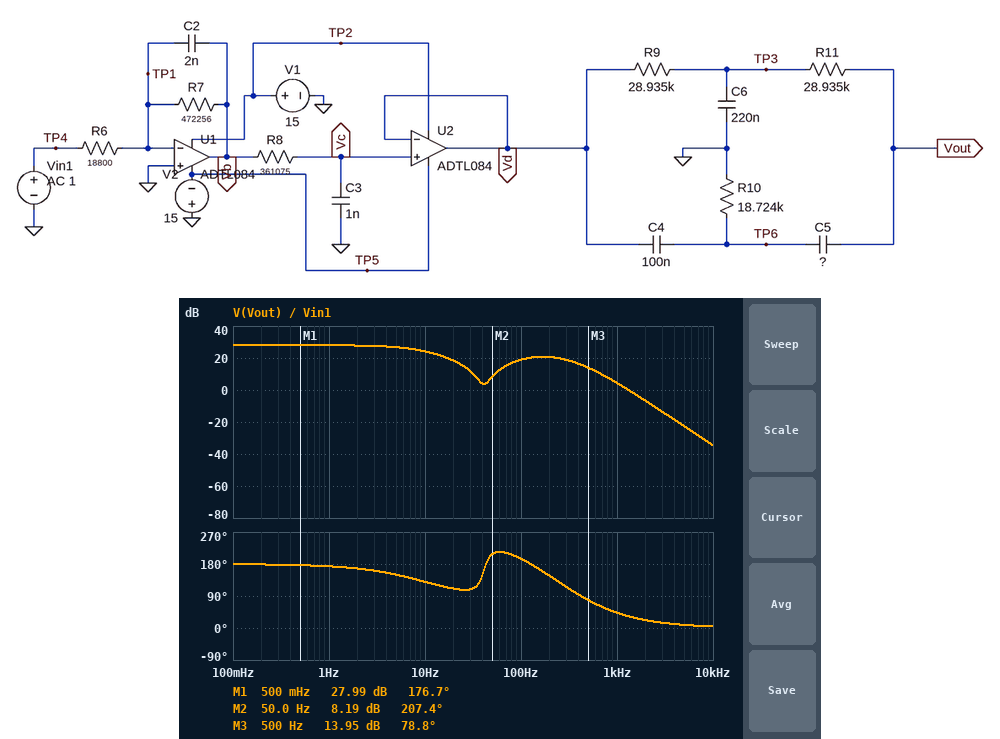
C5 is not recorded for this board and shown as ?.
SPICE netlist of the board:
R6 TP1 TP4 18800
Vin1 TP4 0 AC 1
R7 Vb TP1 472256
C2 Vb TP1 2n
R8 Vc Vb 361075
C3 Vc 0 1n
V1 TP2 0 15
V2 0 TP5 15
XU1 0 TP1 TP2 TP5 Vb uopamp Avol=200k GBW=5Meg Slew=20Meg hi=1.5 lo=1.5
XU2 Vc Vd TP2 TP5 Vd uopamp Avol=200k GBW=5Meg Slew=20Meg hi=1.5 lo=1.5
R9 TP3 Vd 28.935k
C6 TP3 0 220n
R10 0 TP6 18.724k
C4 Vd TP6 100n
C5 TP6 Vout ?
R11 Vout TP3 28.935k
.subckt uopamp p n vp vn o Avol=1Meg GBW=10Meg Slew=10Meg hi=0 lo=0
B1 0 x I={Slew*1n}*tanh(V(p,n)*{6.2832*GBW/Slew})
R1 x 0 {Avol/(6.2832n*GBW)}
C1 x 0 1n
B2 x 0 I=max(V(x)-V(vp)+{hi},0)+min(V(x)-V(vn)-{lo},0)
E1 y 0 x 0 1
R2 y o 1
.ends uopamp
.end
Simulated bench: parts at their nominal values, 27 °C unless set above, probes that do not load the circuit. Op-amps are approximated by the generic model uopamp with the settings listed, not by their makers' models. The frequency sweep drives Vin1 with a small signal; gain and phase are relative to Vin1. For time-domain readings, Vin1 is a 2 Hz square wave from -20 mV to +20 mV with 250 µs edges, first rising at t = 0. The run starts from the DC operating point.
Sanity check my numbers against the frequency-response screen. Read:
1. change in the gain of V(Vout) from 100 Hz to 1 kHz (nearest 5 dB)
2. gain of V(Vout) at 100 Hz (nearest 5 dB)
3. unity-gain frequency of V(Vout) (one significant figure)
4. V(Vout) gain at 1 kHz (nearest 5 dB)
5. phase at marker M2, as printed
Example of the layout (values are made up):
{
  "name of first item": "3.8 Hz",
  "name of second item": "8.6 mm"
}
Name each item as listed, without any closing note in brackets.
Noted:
{
  "change in the gain of V(Vout) from 100 Hz to 1 kHz": "-15 dB",
  "gain of V(Vout) at 100 Hz": "20 dB",
  "unity-gain frequency of V(Vout)": "1 kHz",
  "V(Vout) gain at 1 kHz": "5 dB",
  "phase at marker M2, as printed": "207.4 deg"
}
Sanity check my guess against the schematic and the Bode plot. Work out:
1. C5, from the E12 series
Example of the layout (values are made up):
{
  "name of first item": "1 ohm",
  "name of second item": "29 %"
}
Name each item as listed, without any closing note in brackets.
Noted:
{
  "C5, from the E12 series": "180 nF"
}
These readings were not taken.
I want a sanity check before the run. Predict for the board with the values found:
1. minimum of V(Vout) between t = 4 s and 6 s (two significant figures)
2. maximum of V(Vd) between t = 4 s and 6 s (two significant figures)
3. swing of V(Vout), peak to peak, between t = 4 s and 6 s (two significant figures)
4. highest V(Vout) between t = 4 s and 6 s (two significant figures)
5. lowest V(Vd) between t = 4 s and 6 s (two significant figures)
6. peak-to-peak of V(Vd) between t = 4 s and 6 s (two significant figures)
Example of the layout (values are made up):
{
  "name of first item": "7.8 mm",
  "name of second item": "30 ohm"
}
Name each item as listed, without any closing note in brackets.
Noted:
{
  "minimum of V(Vout) between t = 4 s and 6 s": "-500 mV",
  "maximum of V(Vd) between t = 4 s and 6 s": "500 mV",
  "swing of V(Vout), peak to peak, between t = 4 s and 6 s": "1.0 V",
  "highest V(Vout) between t = 4 s and 6 s": "500 mV",
  "lowest V(Vd) between t = 4 s and 6 s": "-500 mV",
  "peak-to-peak of V(Vd) between t = 4 s and 6 s": "1.0 V"
}
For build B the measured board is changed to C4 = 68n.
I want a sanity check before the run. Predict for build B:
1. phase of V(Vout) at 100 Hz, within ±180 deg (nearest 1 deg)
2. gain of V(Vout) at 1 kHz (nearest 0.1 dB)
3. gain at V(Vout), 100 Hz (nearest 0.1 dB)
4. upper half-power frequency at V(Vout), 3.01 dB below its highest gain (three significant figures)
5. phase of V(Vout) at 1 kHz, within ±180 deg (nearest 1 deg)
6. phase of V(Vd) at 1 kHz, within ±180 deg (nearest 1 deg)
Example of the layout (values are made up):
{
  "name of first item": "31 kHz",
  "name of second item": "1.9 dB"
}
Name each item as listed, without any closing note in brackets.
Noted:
{
  "phase of V(Vout) at 100 Hz, within ±180 deg": "-157 deg",
  "gain of V(Vout) at 1 kHz": "4.3 dB",
  "gain at V(Vout), 100 Hz": "15.9 dB",
  "upper half-power frequency at V(Vout), 3.01 dB below its highest gain": "8.73 Hz",
  "phase of V(Vout) at 1 kHz, within ±180 deg": "47 deg",
  "phase of V(Vd) at 1 kHz, within ±180 deg": "33 deg"
}
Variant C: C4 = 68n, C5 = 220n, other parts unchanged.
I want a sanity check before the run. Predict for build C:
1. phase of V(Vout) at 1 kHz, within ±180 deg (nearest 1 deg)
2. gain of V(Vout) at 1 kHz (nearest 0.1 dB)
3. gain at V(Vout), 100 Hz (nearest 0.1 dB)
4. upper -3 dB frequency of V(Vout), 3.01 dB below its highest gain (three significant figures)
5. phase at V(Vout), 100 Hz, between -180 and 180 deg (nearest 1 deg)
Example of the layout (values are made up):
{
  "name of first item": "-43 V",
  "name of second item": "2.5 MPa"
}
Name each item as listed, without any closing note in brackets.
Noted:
{
  "phase of V(Vout) at 1 kHz, within ±180 deg": "46 deg",
  "gain of V(Vout) at 1 kHz": "4.3 dB",
  "gain at V(Vout), 100 Hz": "16.3 dB",
  "upper -3 dB frequency of V(Vout), 3.01 dB below its highest gain": "7.58 Hz",
  "phase at V(Vout), 100 Hz, between -180 and 180 deg": "-159 deg"
}
